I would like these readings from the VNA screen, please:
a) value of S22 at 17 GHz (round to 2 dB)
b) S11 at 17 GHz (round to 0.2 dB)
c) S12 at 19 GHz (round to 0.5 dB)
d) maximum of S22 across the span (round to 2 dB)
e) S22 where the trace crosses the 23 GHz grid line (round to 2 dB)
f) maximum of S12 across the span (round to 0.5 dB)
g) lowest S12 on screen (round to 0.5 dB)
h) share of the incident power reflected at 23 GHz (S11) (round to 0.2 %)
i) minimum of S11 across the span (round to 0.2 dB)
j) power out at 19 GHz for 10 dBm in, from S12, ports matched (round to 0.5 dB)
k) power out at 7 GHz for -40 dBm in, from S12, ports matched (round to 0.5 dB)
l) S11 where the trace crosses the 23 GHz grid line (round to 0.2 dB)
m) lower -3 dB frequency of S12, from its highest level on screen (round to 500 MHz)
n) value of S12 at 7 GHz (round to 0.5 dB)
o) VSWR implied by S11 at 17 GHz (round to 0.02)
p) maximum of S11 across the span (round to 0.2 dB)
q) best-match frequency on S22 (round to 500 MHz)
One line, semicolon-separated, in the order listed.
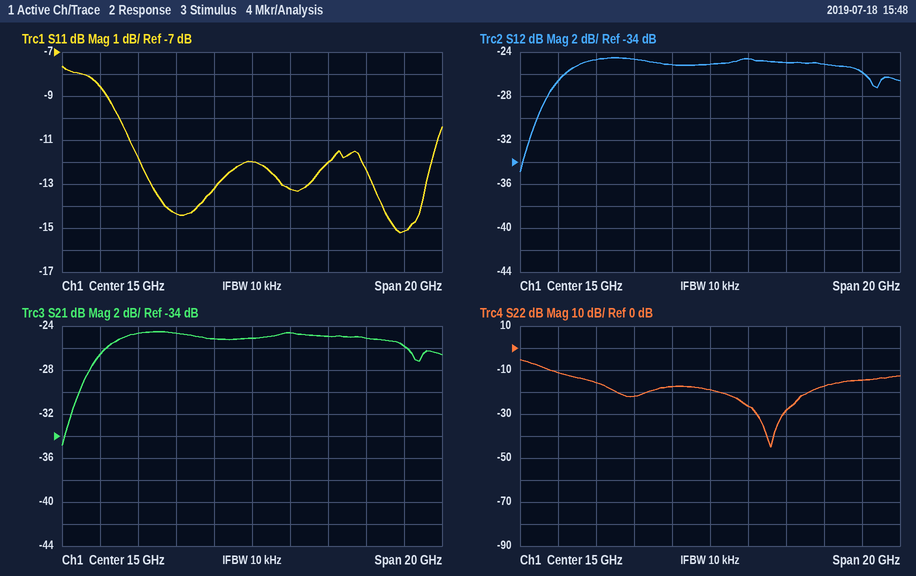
-26 dB; -13.2 dB; -25.0 dB; -6 dB; -14 dB; -24.5 dB; -35.0 dB; 3.0 %; -15.2 dB; -15.0 dBm; -66.5 dBm; -15.2 dB; 6.5 GHz; -26.5 dB; 1.56; -7.6 dB; 18.0 GHz
